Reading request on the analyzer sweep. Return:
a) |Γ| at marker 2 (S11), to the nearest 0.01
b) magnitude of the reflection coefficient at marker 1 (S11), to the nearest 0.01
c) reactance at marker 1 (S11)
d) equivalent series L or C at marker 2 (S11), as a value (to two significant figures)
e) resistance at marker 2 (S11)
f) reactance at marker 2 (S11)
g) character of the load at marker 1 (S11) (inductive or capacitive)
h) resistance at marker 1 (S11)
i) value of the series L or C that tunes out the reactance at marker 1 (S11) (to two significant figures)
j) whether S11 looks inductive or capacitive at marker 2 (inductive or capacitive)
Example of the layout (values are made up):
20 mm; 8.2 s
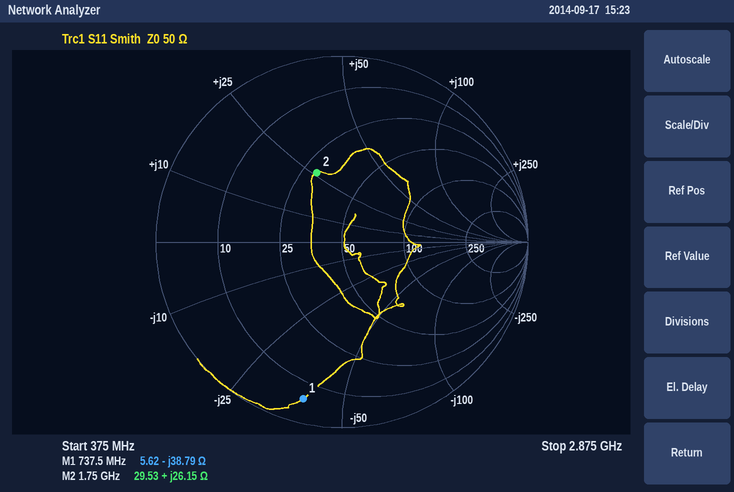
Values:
0.40; 0.87; -38.79 Ω; 2.4 nH; 29.53 Ω; +26.15 Ω; capacitive; 5.62 Ω; 8.4 nH; inductive
